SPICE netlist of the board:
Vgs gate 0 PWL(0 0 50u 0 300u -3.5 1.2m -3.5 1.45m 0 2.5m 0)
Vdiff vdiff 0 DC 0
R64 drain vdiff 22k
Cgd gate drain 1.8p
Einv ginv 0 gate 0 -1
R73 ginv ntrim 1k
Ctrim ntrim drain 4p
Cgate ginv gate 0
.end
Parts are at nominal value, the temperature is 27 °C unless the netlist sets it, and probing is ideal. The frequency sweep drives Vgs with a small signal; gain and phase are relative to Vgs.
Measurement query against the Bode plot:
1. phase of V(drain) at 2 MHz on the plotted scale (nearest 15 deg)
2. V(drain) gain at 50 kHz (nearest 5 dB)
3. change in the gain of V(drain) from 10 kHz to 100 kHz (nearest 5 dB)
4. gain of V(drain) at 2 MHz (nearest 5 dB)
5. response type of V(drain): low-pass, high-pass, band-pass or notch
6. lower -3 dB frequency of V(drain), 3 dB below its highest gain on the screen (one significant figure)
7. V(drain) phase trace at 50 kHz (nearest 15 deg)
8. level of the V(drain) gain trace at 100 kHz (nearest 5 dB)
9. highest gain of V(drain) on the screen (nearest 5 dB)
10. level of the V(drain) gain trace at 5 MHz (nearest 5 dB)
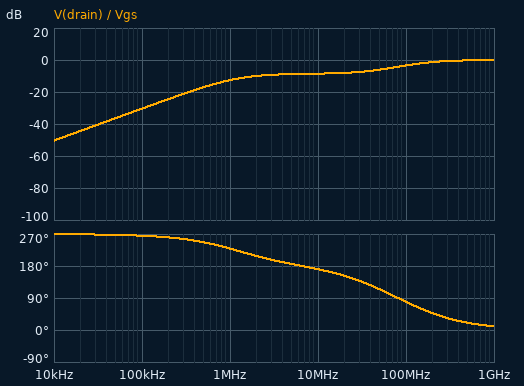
210 deg
-35 dB
20 dB
-10 dB
high-pass
100 MHz
270 deg
-30 dB
0 dB
-10 dB
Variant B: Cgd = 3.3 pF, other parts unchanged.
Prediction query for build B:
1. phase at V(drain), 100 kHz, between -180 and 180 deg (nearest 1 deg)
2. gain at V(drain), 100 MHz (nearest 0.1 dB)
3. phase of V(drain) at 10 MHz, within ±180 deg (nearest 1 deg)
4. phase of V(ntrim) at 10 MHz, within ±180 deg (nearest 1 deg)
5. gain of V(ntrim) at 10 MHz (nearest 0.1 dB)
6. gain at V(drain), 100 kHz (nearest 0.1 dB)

-97 deg
-2.5 dB
129 deg
167 deg
0 dB
-40.3 dB
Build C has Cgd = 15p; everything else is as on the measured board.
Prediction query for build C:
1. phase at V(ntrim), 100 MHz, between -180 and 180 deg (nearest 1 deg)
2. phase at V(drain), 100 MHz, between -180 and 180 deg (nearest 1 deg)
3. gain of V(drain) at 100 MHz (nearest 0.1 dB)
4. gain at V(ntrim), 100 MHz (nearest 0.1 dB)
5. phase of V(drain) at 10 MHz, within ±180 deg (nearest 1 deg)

54 deg
11 deg
-0.6 dB
0 dB
10 deg
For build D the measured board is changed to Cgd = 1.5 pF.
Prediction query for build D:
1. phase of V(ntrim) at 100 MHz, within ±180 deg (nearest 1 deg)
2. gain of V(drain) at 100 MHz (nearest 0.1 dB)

112 deg
-3.5 dB
